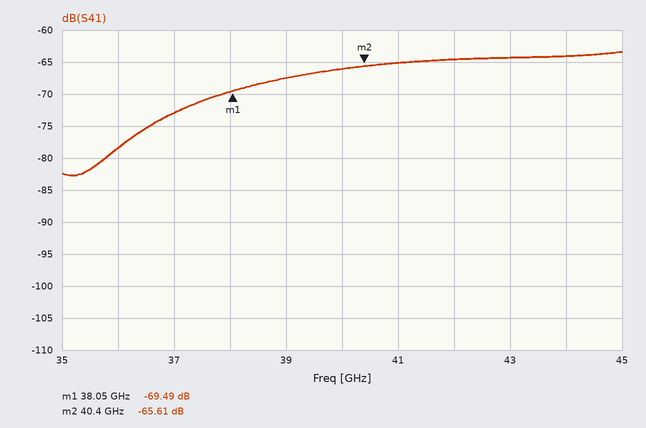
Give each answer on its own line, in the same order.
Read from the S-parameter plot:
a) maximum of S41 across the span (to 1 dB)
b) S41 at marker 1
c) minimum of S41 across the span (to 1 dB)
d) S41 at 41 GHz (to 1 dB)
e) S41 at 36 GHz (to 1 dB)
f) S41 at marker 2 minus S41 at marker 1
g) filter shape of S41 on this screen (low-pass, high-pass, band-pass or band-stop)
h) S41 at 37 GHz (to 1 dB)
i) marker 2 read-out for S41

-63 dB
-69.49 dB
-83 dB
-65 dB
-78 dB
3.88 dB
high-pass
-73 dB
-65.61 dB
